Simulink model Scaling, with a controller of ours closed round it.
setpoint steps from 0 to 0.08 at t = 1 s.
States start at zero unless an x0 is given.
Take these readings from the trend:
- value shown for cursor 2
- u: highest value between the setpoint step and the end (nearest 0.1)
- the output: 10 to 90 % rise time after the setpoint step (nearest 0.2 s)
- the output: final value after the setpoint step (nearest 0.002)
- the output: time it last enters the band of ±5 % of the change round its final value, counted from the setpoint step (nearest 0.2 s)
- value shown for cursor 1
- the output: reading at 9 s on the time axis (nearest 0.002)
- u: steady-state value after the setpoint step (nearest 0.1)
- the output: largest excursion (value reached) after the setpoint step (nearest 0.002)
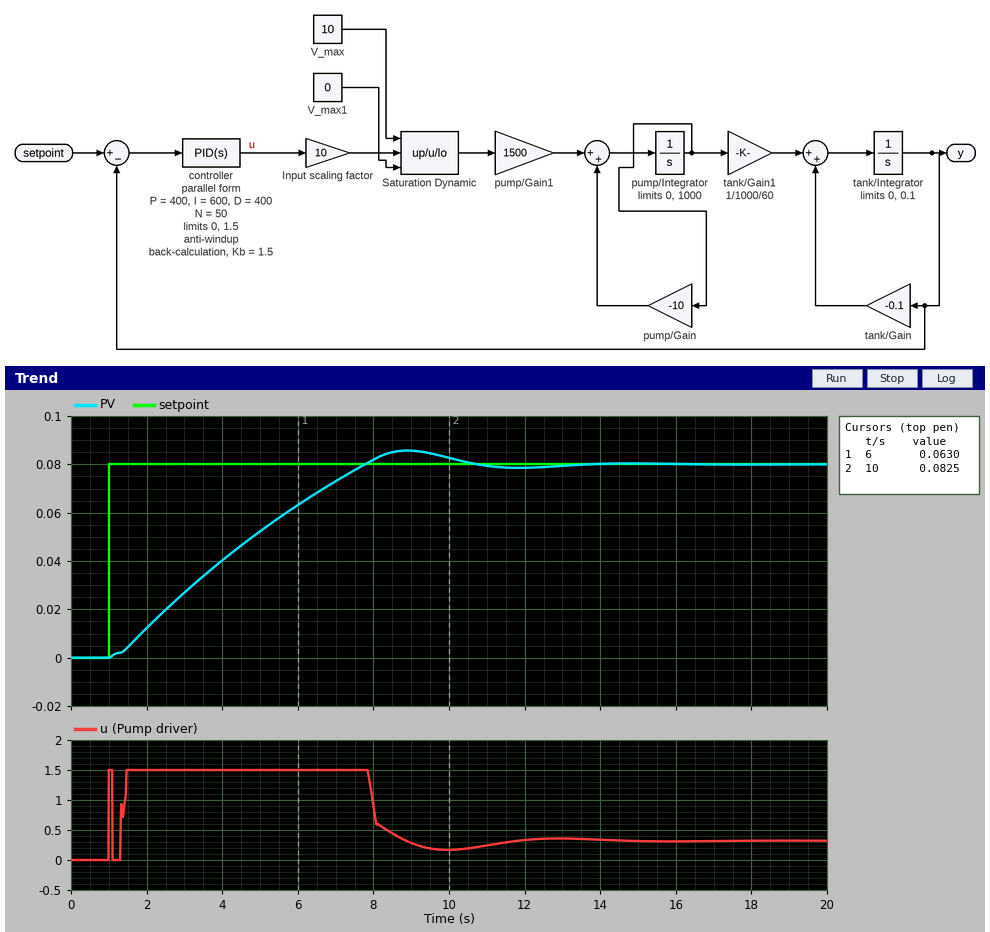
0.0825
1.5
5.2 s
0.080
8.6 s
0.0630
0.086
0.3
0.086
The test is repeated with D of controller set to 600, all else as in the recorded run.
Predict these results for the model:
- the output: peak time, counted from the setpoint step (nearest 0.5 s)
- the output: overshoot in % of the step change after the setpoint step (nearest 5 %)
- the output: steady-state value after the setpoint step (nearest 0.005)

8.5 s
10 %
0.080
